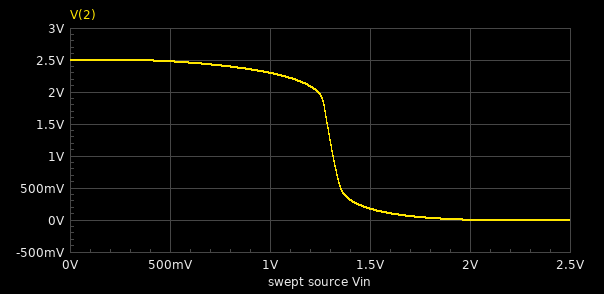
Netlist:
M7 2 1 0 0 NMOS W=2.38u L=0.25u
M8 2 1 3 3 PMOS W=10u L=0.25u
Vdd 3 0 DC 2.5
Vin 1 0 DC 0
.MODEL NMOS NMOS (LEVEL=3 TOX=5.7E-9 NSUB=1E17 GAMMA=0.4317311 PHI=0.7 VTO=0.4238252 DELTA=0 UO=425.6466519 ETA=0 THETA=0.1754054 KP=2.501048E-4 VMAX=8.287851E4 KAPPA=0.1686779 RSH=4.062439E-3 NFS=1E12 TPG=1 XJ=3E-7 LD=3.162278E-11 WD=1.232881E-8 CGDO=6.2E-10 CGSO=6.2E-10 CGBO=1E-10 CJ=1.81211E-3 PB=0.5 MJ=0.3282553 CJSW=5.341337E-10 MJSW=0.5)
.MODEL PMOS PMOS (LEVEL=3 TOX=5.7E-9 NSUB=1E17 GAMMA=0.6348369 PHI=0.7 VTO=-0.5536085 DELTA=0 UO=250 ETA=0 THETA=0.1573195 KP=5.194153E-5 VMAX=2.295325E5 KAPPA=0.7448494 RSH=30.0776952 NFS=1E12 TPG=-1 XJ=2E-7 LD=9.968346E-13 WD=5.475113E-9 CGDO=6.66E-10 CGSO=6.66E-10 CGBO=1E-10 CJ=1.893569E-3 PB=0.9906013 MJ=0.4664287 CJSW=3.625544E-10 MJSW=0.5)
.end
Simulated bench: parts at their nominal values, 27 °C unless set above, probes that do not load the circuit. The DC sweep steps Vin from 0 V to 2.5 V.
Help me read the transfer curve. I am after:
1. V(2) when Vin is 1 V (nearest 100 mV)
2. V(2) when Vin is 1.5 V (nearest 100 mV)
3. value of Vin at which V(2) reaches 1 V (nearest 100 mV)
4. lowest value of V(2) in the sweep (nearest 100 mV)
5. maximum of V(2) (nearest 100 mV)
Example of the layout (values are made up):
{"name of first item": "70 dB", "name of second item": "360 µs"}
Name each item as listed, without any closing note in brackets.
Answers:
{"V(2) when Vin is 1 V": "2.3 V", "V(2) when Vin is 1.5 V": "200 mV", "value of Vin at which V(2) reaches 1 V": "1.3 V", "lowest value of V(2) in the sweep": "0 V", "maximum of V(2)": "2.5 V"}
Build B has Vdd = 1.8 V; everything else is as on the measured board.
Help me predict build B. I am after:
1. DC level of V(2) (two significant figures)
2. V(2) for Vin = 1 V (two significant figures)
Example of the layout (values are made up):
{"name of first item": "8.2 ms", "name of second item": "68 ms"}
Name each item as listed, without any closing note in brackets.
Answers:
{"DC level of V(2)": "1.8 V", "V(2) for Vin = 1 V": "130 mV"}
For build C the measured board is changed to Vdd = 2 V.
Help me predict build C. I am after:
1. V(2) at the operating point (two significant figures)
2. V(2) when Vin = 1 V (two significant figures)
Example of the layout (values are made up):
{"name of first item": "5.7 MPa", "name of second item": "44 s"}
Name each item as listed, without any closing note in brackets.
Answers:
{"V(2) at the operating point": "2.0 V", "V(2) when Vin = 1 V": "1.1 V"}
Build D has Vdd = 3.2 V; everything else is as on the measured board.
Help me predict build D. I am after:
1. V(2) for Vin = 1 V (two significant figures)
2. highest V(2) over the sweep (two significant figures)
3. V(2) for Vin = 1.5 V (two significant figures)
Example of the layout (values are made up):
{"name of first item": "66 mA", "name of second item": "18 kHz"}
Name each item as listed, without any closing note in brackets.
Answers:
{"V(2) for Vin = 1 V": "3.1 V", "highest V(2) over the sweep": "3.2 V", "V(2) for Vin = 1.5 V": "2.8 V"}
